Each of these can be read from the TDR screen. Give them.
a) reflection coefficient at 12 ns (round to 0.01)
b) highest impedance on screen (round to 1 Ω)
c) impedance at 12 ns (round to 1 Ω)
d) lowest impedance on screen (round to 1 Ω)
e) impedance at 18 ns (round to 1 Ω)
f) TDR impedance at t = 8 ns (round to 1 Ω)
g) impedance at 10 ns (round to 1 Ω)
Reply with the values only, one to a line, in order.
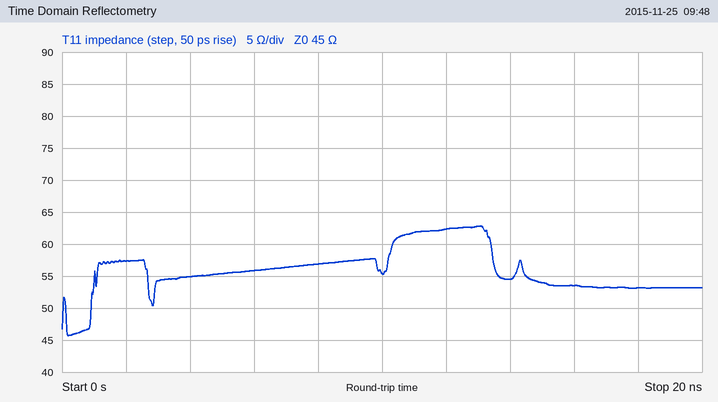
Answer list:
+0.16
63 Ω
62 Ω
46 Ω
53 Ω
57 Ω
55 Ω
